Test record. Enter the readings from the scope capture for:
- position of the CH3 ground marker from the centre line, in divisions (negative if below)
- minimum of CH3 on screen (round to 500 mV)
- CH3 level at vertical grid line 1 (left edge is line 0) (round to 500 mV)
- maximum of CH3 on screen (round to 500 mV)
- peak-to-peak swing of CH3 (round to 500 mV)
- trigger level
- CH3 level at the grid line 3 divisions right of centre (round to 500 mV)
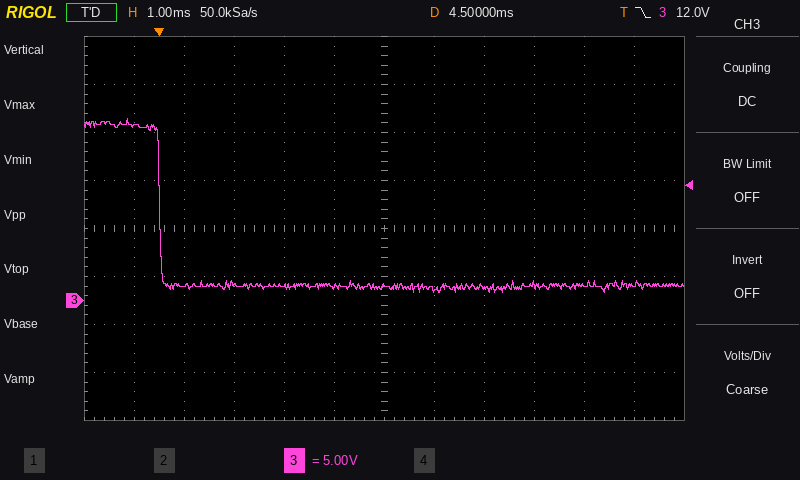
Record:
-1.5 div
1.0 V
18.0 V
19.0 V
18.0 V
12.0 V
1.5 V
